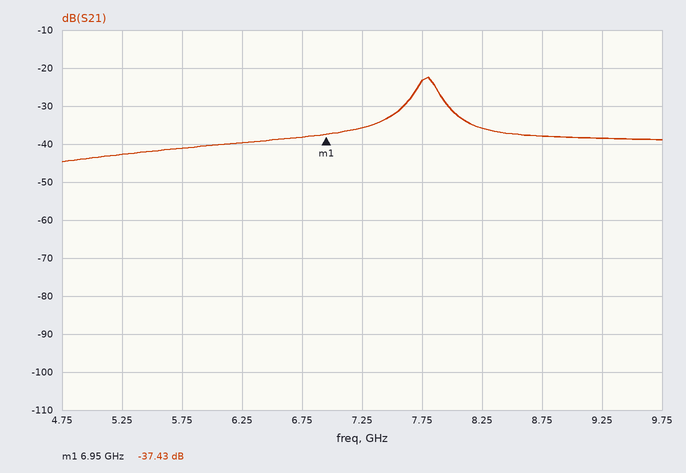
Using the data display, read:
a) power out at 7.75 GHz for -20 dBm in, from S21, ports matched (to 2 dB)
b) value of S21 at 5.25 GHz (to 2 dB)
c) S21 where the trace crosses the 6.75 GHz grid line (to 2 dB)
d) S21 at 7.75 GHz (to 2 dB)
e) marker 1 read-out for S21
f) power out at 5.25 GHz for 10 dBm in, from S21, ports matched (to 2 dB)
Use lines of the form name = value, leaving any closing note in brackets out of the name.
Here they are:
power out at 7.75 GHz for -20 dBm in, from S21, ports matched = -44 dBm
value of S21 at 5.25 GHz = -42 dB
S21 where the trace crosses the 6.75 GHz grid line = -38 dB
S21 at 7.75 GHz = -24 dB
marker 1 read-out for S21 = -37.43 dB
power out at 5.25 GHz for 10 dBm in, from S21, ports matched = -32 dBm
